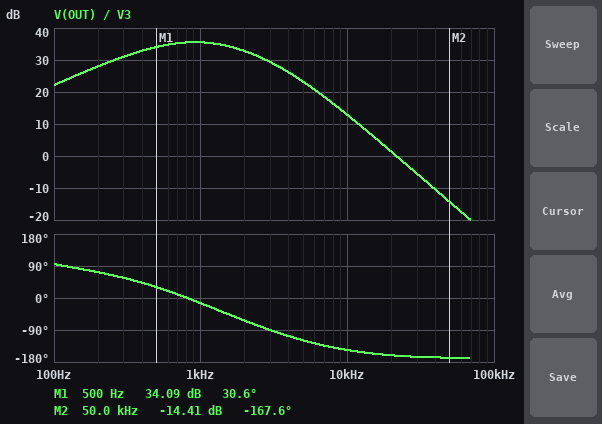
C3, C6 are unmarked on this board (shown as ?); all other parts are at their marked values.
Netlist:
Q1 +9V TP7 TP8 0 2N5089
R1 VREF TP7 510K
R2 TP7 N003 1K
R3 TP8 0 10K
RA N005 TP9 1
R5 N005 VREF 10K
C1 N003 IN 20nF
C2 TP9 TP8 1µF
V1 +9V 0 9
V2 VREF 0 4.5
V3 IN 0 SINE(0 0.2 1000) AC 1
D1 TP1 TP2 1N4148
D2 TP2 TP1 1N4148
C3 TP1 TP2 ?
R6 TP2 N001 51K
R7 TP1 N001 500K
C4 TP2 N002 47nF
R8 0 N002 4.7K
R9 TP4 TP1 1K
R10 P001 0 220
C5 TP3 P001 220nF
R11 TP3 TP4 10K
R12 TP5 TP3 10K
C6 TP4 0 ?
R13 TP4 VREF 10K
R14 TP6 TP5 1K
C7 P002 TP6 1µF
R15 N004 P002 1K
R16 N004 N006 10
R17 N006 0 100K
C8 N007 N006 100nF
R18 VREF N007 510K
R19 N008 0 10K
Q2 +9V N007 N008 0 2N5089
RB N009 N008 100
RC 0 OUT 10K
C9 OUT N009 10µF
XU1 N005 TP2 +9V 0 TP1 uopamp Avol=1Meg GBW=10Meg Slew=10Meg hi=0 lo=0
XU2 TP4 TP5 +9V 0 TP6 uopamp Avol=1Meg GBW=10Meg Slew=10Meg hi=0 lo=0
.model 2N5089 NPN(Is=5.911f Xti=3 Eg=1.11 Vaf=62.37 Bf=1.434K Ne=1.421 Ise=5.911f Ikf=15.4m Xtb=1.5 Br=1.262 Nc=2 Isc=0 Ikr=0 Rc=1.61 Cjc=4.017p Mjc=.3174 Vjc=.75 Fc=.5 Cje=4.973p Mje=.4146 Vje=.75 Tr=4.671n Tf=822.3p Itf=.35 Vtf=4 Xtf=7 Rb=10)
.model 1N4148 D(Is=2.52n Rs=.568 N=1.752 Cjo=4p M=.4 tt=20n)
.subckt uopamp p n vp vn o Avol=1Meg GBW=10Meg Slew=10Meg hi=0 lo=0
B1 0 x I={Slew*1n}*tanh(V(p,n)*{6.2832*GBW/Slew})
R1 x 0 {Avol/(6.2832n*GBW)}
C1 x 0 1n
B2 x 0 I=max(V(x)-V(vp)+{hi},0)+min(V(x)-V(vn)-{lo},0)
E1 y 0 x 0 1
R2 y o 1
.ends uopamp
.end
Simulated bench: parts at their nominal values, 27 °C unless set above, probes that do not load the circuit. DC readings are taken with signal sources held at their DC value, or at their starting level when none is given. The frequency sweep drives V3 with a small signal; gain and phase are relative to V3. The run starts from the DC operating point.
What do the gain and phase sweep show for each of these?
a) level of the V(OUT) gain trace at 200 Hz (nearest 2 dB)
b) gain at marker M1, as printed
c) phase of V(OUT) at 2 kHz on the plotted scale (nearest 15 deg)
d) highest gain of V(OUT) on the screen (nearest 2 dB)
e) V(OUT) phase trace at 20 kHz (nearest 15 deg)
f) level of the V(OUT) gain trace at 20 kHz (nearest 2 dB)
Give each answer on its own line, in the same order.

28 dB
34.09 dB
-60 deg
36 dB
-165 deg
2 dB
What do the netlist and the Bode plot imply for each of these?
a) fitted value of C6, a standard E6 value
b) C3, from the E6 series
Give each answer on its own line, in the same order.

150 nF
68 pF
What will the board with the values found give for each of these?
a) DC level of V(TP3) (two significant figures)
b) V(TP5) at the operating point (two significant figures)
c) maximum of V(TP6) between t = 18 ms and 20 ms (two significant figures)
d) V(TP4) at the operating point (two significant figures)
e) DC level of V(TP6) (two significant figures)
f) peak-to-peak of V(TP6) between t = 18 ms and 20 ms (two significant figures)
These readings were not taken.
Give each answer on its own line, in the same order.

4.5 V
4.5 V
5.0 V
4.5 V
4.5 V
980 mV
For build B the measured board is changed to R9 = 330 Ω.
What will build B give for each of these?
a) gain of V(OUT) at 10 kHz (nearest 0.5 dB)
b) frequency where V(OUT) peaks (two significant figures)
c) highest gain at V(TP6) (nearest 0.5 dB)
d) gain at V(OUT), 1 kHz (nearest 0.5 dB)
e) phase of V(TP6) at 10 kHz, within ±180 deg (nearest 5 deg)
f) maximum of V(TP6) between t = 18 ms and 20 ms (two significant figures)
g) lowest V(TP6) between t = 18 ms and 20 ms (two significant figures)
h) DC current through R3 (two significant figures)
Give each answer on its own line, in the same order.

22.0 dB
1.3 kHz
39.0 dB
38.5 dB
-135 deg
5.1 V
3.9 V
360 µA
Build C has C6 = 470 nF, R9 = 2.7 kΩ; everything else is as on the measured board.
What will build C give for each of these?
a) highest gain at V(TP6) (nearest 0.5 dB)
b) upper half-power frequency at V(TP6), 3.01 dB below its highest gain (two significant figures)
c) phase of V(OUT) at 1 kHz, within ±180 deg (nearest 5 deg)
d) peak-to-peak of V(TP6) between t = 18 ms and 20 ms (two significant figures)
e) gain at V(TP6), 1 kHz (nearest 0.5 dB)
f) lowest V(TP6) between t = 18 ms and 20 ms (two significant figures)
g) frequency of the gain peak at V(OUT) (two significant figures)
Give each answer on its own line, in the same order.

24.0 dB
1.0 kHz
-55 deg
210 mV
21.5 dB
4.4 V
390 Hz
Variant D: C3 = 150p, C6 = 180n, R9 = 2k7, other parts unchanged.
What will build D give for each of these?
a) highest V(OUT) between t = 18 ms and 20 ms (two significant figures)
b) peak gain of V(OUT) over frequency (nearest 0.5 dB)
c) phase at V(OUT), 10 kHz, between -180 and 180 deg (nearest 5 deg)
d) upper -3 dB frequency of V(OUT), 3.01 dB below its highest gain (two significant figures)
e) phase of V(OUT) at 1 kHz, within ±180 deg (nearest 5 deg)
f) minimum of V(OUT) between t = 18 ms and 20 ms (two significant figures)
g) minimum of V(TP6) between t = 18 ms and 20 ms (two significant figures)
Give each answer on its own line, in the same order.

230 mV
29.5 dB
-160 deg
1.2 kHz
-55 deg
-230 mV
4.3 V
